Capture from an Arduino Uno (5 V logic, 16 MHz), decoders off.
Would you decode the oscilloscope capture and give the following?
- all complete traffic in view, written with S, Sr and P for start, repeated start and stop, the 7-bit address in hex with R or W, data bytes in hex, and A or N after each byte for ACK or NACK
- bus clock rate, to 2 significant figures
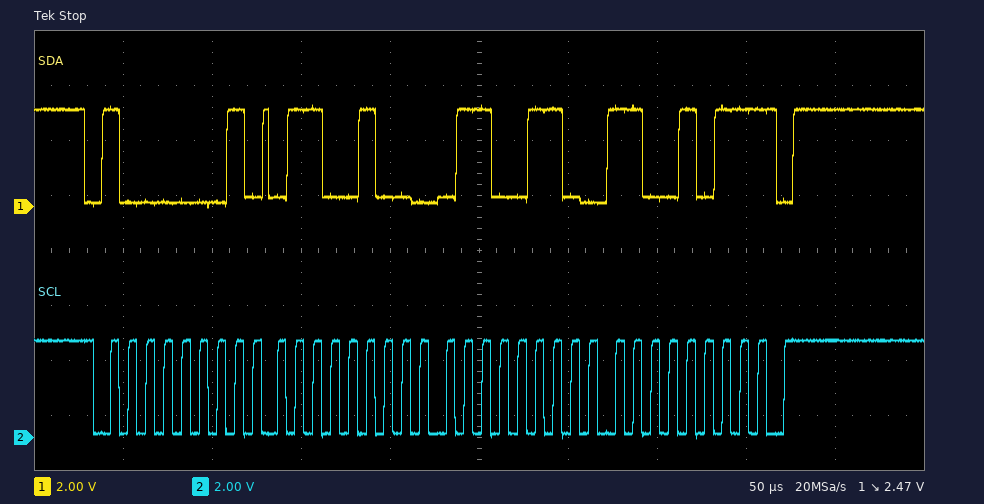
S 40R A 64 A 66 A CB N P
100 kHz
